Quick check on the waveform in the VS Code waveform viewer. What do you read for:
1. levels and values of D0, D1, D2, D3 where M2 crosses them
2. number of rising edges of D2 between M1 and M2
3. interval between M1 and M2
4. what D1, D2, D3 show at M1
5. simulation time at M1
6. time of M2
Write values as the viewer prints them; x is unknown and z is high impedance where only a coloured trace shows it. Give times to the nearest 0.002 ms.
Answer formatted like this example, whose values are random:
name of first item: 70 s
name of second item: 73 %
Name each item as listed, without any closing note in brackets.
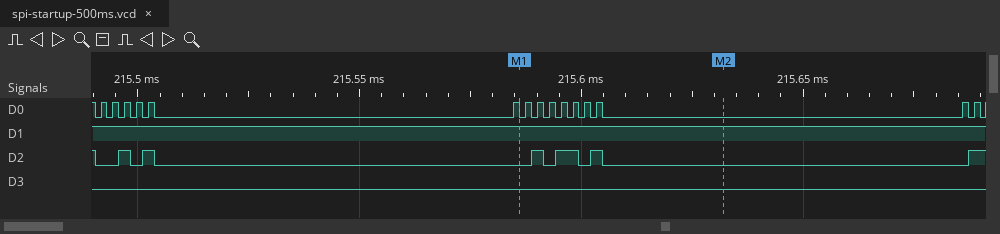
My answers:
levels and values of D0, D1, D2, D3 where M2 crosses them: D0=0, D1=1, D2=0, D3=0
number of rising edges of D2 between M1 and M2: 3
interval between M1 and M2: 0.046 ms
what D1, D2, D3 show at M1: D1=1, D2=0, D3=0
simulation time at M1: 215.586 ms
time of M2: 215.632 ms
